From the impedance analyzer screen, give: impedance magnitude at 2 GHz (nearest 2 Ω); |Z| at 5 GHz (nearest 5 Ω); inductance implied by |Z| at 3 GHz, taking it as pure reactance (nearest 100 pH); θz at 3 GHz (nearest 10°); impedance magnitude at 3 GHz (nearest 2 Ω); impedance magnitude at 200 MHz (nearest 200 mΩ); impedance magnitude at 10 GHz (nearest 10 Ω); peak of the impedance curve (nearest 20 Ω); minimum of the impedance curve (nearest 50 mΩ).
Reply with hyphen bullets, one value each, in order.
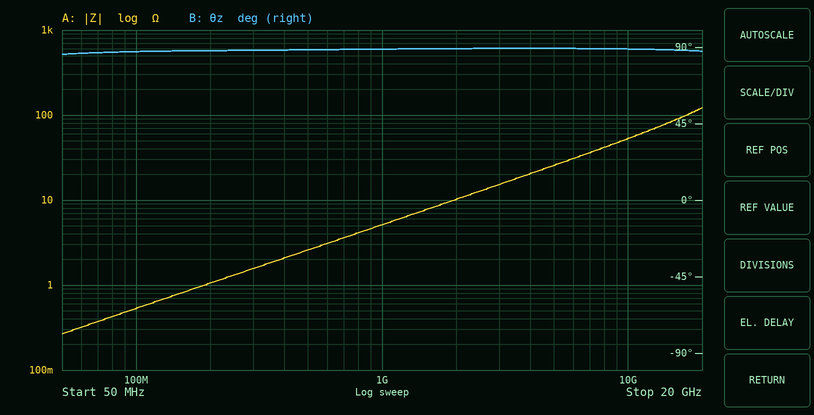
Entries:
- 10 Ω
- 25 Ω
- 800 pH
- 90°
- 16 Ω
- 1.0 Ω
- 50 Ω
- 120 Ω
- 250 mΩ
